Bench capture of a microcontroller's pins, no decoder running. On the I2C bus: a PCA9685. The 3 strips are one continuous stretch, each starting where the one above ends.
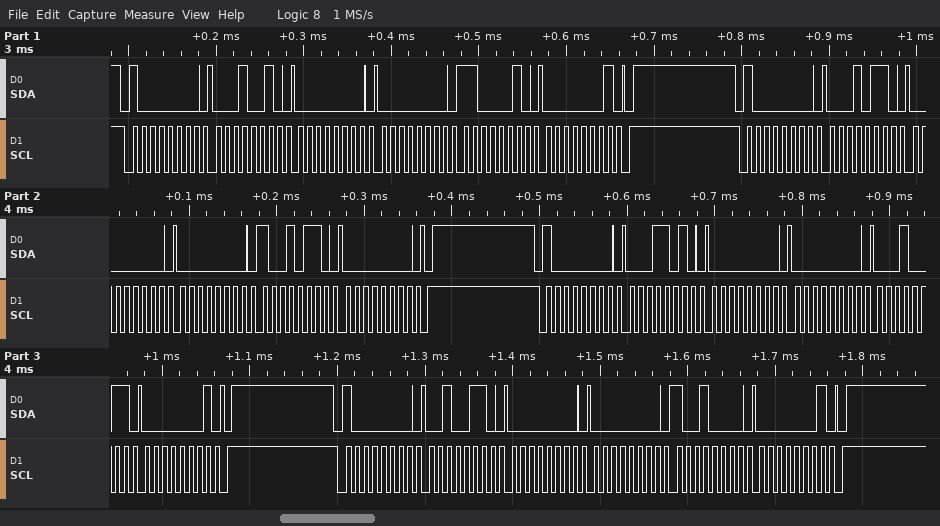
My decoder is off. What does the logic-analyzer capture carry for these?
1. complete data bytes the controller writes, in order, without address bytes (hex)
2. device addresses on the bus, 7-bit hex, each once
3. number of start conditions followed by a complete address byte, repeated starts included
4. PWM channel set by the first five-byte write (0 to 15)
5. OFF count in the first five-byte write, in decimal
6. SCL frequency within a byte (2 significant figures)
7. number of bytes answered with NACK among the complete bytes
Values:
12 00 00 C2 01 16 00 00 96 00 1A 00 00 13 01 26 00 00 90 01
0x40
4
3
450
100 kHz
0
